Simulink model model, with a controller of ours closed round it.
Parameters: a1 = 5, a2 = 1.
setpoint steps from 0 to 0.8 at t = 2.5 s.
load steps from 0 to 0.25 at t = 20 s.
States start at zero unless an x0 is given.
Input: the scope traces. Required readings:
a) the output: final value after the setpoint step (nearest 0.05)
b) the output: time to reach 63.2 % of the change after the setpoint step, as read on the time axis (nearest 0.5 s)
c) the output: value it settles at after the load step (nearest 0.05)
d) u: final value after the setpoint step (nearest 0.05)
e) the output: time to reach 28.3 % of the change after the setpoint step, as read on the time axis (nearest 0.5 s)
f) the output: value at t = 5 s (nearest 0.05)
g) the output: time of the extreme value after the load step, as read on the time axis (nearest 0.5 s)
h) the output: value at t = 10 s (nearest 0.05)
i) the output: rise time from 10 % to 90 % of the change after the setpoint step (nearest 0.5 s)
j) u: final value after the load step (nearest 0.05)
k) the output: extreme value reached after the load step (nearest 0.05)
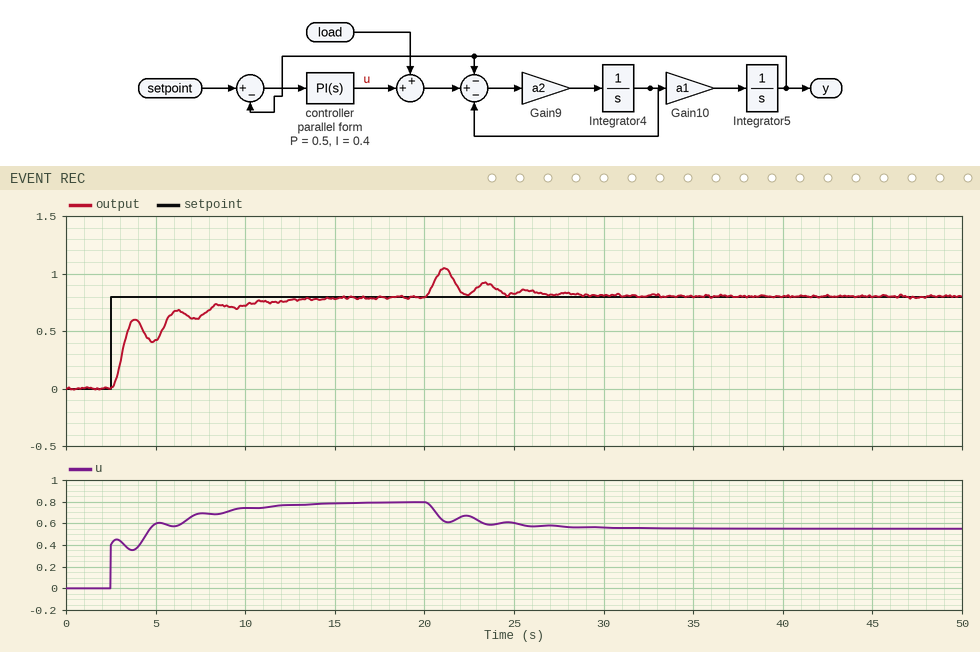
0.80
3.5 s
0.80
0.80
3.0 s
0.40
21.0 s
0.70
5.5 s
0.55
1.05
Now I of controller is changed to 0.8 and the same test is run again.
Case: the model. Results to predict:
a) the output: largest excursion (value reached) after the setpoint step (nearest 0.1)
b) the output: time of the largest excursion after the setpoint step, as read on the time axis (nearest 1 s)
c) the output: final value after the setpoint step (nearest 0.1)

0.9
6 s
0.8
